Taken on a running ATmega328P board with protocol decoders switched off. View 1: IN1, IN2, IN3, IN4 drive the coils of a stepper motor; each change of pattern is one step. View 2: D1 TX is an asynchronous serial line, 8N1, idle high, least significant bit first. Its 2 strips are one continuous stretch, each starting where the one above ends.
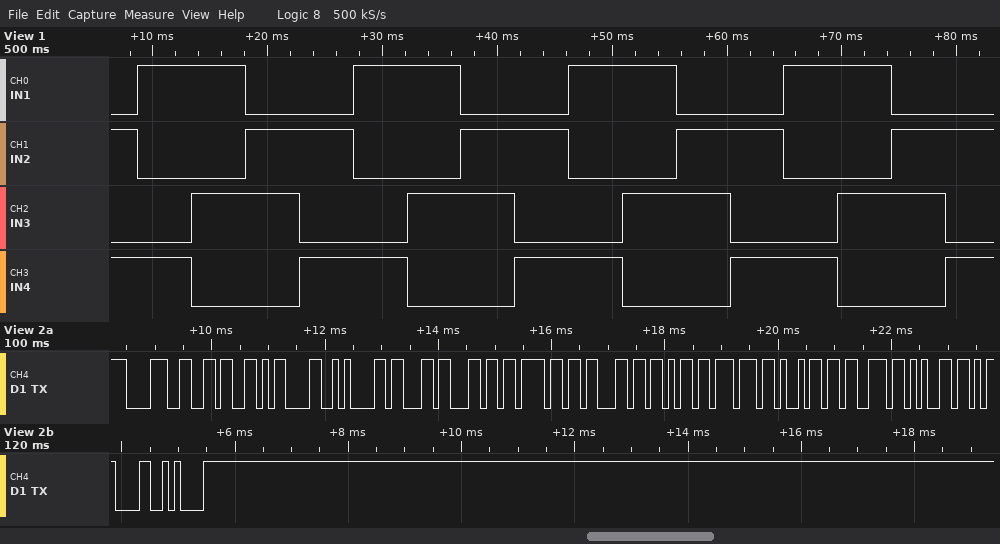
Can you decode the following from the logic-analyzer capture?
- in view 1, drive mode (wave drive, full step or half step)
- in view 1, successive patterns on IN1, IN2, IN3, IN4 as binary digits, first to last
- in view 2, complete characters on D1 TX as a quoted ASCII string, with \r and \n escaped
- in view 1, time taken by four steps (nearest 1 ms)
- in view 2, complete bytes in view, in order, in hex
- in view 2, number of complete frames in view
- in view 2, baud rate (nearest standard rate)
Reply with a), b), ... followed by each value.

a) full step
b) 0101 1001 1010 0110 0101 1001 1010 0110 0101 1001 1010 0110 0101 1001 1010 0110 0101
c) "86\r\nclockwise\r\n"
d) 19 ms
e) 38 36 0D 0A 63 6C 6F 63 6B 77 69 73 65 0D 0A
f) 15
g) 9600 baud
